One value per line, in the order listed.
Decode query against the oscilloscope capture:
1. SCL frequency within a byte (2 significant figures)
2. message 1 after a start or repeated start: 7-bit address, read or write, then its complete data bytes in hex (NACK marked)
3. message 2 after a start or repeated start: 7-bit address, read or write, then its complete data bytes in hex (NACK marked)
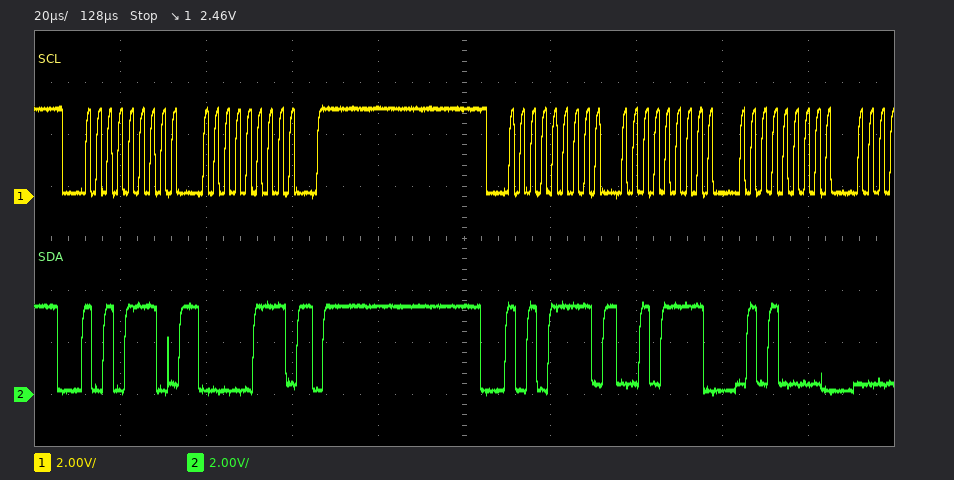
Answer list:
400 kHz
0x57 write: 07
0x57 read: 2F 50
